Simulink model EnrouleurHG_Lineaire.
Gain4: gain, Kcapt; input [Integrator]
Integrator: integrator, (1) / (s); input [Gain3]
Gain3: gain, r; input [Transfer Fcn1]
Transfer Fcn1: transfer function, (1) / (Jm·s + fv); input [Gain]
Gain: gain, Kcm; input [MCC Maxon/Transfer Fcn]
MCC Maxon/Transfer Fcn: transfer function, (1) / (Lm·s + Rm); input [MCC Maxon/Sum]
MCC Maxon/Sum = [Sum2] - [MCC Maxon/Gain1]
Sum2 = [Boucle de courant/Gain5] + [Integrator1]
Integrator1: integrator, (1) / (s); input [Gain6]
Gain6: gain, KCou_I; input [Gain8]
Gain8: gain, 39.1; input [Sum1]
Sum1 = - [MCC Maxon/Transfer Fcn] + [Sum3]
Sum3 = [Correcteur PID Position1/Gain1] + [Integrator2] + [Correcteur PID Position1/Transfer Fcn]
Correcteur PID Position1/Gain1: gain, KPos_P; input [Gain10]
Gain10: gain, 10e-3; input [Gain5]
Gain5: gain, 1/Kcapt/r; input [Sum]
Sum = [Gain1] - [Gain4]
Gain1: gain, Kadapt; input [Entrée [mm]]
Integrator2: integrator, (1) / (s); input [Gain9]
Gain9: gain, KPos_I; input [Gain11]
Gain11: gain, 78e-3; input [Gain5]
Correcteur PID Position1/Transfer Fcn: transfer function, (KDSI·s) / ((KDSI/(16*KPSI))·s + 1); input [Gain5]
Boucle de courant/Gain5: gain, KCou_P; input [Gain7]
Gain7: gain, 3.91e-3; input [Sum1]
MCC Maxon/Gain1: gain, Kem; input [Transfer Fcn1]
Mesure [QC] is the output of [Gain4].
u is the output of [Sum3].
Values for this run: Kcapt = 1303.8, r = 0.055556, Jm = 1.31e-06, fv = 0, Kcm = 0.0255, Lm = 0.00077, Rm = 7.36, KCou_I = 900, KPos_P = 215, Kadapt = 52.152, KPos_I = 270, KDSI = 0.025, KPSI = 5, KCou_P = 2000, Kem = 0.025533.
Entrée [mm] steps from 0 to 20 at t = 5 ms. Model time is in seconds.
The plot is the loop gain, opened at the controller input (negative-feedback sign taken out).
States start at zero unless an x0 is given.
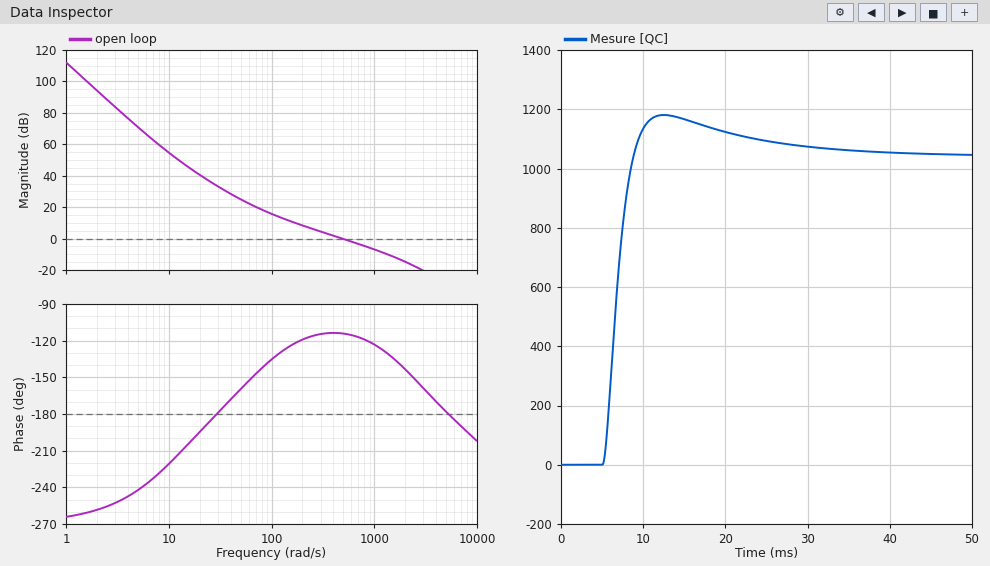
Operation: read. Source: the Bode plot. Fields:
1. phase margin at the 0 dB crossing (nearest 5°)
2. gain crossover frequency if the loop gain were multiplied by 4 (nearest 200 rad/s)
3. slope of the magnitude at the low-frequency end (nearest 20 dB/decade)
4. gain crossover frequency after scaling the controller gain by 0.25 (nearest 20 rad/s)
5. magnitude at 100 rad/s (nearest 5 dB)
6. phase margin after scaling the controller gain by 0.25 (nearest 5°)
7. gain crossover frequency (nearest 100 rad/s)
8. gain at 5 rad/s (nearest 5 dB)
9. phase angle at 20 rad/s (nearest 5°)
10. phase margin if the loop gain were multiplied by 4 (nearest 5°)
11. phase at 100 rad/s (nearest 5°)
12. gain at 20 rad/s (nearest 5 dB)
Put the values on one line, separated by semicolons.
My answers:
65°; 1600 rad/s; -60 dB/decade; 140 rad/s; 15 dB; 55°; 500 rad/s; 70 dB; -195°; 45°; -135°; 40 dB
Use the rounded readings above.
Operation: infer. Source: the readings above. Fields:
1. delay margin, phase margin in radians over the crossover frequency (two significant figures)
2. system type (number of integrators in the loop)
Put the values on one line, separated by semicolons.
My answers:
0.0023 s; 3
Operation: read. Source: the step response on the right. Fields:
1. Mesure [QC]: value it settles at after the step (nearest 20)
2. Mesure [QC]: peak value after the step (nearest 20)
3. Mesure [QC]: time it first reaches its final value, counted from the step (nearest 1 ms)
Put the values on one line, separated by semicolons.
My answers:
1040; 1180; 4 ms
